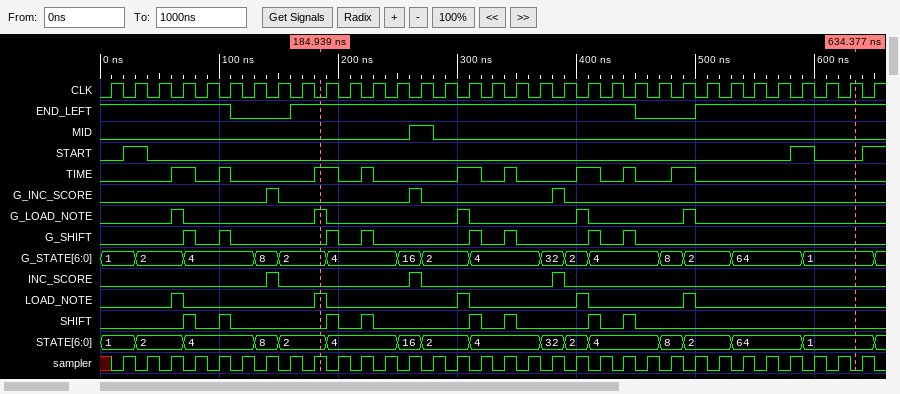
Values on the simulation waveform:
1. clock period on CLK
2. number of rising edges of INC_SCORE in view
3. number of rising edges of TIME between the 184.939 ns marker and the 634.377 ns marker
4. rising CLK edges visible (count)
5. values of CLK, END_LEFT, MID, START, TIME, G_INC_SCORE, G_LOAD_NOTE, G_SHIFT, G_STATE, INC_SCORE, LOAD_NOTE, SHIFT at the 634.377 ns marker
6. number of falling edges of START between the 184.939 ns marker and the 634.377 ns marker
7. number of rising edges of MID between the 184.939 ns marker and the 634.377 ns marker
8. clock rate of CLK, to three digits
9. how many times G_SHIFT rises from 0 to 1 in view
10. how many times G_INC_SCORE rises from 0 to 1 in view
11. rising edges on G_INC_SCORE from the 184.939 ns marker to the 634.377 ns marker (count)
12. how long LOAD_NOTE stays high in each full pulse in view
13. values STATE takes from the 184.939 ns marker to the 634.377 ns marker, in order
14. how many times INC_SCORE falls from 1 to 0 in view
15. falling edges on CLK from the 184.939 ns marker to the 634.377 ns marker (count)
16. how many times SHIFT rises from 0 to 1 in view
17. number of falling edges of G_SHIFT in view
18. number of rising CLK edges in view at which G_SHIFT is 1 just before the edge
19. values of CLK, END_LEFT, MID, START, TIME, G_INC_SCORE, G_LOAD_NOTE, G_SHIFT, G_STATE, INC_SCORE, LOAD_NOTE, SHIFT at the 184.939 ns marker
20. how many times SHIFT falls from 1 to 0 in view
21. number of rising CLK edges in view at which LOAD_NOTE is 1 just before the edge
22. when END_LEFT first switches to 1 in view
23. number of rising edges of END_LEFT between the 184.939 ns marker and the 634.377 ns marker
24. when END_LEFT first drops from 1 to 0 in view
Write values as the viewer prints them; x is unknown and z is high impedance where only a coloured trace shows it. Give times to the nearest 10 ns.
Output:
20 ns
3
6
33
CLK=1, END_LEFT=1, MID=0, START=0, TIME=0, G_INC_SCORE=0, G_LOAD_NOTE=0, G_SHIFT=0, G_STATE=1, INC_SCORE=0, LOAD_NOTE=0, SHIFT=0
1
1
50.0 MHz
8
3
2
10 ns, 10 ns, 10 ns, 10 ns, 10 ns
2, 4, 16, 2, 4, 32, 2, 4, 8, 2, 64, 1
3
22
8
8
4
CLK=0, END_LEFT=1, MID=0, START=0, TIME=1, G_INC_SCORE=0, G_LOAD_NOTE=1, G_SHIFT=0, G_STATE=2, INC_SCORE=0, LOAD_NOTE=1, SHIFT=0
8
4
160 ns
1
110 ns
